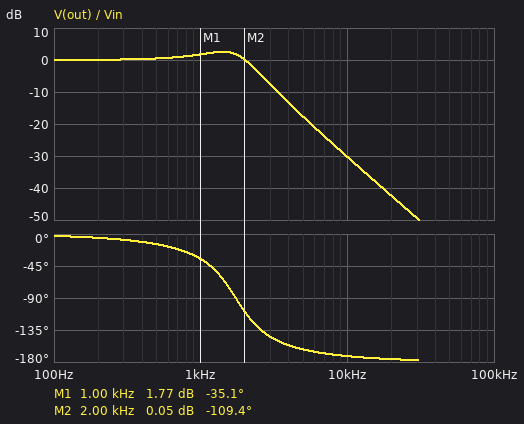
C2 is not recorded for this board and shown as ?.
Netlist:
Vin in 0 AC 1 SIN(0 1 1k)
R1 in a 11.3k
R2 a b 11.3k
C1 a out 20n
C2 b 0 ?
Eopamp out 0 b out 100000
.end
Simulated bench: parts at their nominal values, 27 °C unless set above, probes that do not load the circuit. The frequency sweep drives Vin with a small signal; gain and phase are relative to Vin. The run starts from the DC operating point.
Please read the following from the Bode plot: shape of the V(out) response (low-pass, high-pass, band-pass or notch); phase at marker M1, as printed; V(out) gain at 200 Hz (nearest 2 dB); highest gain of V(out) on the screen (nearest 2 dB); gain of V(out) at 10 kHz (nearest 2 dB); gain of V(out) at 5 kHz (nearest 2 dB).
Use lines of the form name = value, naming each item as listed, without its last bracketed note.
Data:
shape of the V(out) response = low-pass
phase at marker M1, as printed = -35.1 deg
V(out) gain at 200 Hz = 0 dB
highest gain of V(out) on the screen = 2 dB
gain of V(out) at 10 kHz = -30 dB
gain of V(out) at 5 kHz = -18 dB
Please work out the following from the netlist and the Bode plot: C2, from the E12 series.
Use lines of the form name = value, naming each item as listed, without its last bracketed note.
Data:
C2, from the E12 series = 3.3 nF
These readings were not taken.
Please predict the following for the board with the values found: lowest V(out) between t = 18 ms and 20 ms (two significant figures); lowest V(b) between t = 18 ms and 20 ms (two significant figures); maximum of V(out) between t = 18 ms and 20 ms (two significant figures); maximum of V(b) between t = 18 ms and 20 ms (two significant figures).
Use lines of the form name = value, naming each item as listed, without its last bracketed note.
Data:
lowest V(out) between t = 18 ms and 20 ms = -1.2 V
lowest V(b) between t = 18 ms and 20 ms = -1.2 V
maximum of V(out) between t = 18 ms and 20 ms = 1.2 V
maximum of V(b) between t = 18 ms and 20 ms = 1.2 V
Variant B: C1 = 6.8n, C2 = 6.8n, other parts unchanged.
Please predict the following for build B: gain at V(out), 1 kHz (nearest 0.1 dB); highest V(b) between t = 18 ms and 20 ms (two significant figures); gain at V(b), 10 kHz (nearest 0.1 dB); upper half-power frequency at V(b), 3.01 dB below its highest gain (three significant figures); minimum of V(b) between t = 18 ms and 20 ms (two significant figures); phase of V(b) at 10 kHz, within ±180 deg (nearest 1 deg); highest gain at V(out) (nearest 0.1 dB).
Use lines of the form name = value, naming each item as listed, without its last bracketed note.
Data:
gain at V(out), 1 kHz = -1.8 dB
highest V(b) between t = 18 ms and 20 ms = 810 mV
gain at V(b), 10 kHz = -27.7 dB
upper half-power frequency at V(b), 3.01 dB below its highest gain = 1.33 kHz
minimum of V(b) between t = 18 ms and 20 ms = -810 mV
phase of V(b) at 10 kHz, within ±180 deg = -157 deg
highest gain at V(out) = 0 dB
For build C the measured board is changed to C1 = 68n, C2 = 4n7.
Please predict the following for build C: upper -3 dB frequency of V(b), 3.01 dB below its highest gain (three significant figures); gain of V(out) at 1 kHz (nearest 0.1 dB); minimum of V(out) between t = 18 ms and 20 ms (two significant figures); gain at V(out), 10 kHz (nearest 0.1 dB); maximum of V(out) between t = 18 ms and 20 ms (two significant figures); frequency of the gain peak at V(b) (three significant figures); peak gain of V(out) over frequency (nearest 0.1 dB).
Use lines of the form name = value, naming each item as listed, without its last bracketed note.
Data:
upper -3 dB frequency of V(b), 3.01 dB below its highest gain = 922 Hz
gain of V(out) at 1 kHz = 0.9 dB
minimum of V(out) between t = 18 ms and 20 ms = -1.1 V
gain at V(out), 10 kHz = -44.1 dB
maximum of V(out) between t = 18 ms and 20 ms = 1.1 V
frequency of the gain peak at V(b) = 731 Hz
peak gain of V(out) over frequency = 5.9 dB
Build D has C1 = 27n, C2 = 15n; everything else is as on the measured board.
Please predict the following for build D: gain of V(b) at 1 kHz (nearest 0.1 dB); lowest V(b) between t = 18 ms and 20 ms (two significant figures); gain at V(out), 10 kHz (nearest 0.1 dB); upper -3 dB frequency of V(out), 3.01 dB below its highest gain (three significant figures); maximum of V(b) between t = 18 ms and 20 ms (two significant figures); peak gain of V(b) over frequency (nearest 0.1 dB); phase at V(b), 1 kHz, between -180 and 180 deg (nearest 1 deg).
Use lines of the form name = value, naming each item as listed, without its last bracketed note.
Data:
gain of V(b) at 1 kHz = -7.5 dB
lowest V(b) between t = 18 ms and 20 ms = -420 mV
gain at V(out), 10 kHz = -46.2 dB
upper -3 dB frequency of V(out), 3.01 dB below its highest gain = 662 Hz
maximum of V(b) between t = 18 ms and 20 ms = 420 mV
peak gain of V(b) over frequency = 0 dB
phase at V(b), 1 kHz, between -180 and 180 deg = -116 deg
